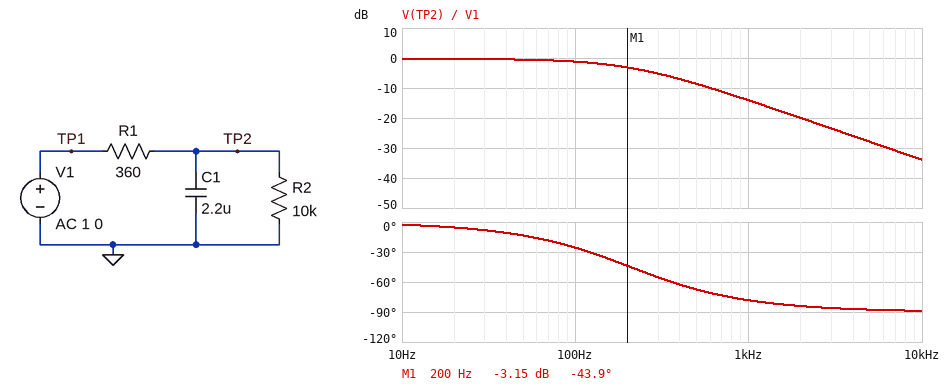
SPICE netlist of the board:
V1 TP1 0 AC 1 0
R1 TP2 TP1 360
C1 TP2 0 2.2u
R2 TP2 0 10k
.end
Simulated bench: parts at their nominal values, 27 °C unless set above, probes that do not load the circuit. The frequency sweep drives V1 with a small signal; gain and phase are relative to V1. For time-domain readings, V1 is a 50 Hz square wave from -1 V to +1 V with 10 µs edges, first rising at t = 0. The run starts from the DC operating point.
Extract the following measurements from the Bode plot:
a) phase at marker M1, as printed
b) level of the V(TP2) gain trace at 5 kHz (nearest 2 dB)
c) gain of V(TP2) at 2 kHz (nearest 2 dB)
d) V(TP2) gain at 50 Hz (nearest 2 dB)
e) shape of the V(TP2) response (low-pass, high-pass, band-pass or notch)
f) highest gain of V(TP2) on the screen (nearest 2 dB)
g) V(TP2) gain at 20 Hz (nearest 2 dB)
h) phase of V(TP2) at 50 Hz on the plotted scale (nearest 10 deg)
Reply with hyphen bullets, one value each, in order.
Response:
- -43.9 deg
- -28 dB
- -20 dB
- 0 dB
- low-pass
- 0 dB
- 0 dB
- -10 deg
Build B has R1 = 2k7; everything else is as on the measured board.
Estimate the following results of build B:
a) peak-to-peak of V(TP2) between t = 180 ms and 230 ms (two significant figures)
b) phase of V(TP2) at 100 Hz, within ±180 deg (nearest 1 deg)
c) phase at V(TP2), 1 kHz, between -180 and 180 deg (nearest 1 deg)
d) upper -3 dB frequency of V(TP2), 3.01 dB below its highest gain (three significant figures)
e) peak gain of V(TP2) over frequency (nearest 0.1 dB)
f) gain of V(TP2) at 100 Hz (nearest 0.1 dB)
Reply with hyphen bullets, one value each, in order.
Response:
- 1.2 V
- -71 deg
- -88 deg
- 34.0 Hz
- -2.1 dB
- -11.9 dB
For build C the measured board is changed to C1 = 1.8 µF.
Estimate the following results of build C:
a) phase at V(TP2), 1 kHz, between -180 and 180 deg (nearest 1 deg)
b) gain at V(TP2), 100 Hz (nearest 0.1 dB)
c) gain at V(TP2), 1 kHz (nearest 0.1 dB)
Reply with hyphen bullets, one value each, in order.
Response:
- -76 deg
- -0.9 dB
- -12.5 dB
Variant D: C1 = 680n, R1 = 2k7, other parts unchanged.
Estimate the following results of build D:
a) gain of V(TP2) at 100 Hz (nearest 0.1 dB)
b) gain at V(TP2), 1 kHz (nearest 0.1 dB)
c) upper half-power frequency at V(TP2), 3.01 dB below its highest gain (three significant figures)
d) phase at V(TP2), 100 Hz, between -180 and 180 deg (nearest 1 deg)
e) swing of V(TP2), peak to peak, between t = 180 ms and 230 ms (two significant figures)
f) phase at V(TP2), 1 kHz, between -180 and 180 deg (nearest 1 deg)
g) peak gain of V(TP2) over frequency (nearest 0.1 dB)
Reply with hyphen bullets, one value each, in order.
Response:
- -4.7 dB
- -21.3 dB
- 110 Hz
- -42 deg
- 1.6 V
- -84 deg
- -2.1 dB
